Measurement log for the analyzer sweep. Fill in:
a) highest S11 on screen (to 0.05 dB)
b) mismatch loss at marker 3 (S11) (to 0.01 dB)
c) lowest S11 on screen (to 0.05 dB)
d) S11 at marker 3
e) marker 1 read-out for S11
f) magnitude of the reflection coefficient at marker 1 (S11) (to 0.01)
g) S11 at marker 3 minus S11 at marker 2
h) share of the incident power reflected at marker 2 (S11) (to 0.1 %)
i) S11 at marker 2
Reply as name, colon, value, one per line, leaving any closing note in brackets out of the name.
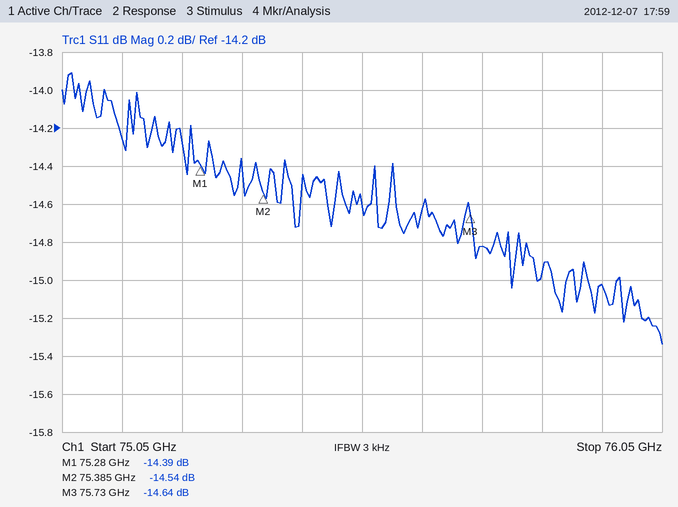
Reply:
highest S11 on screen: -13.90 dB
mismatch loss at marker 3 (S11): 0.15 dB
lowest S11 on screen: -15.35 dB
S11 at marker 3: -14.64 dB
marker 1 read-out for S11: -14.39 dB
magnitude of the reflection coefficient at marker 1 (S11): 0.19
S11 at marker 3 minus S11 at marker 2: -0.10 dB
share of the incident power reflected at marker 2 (S11): 3.5 %
S11 at marker 2: -14.54 dB
